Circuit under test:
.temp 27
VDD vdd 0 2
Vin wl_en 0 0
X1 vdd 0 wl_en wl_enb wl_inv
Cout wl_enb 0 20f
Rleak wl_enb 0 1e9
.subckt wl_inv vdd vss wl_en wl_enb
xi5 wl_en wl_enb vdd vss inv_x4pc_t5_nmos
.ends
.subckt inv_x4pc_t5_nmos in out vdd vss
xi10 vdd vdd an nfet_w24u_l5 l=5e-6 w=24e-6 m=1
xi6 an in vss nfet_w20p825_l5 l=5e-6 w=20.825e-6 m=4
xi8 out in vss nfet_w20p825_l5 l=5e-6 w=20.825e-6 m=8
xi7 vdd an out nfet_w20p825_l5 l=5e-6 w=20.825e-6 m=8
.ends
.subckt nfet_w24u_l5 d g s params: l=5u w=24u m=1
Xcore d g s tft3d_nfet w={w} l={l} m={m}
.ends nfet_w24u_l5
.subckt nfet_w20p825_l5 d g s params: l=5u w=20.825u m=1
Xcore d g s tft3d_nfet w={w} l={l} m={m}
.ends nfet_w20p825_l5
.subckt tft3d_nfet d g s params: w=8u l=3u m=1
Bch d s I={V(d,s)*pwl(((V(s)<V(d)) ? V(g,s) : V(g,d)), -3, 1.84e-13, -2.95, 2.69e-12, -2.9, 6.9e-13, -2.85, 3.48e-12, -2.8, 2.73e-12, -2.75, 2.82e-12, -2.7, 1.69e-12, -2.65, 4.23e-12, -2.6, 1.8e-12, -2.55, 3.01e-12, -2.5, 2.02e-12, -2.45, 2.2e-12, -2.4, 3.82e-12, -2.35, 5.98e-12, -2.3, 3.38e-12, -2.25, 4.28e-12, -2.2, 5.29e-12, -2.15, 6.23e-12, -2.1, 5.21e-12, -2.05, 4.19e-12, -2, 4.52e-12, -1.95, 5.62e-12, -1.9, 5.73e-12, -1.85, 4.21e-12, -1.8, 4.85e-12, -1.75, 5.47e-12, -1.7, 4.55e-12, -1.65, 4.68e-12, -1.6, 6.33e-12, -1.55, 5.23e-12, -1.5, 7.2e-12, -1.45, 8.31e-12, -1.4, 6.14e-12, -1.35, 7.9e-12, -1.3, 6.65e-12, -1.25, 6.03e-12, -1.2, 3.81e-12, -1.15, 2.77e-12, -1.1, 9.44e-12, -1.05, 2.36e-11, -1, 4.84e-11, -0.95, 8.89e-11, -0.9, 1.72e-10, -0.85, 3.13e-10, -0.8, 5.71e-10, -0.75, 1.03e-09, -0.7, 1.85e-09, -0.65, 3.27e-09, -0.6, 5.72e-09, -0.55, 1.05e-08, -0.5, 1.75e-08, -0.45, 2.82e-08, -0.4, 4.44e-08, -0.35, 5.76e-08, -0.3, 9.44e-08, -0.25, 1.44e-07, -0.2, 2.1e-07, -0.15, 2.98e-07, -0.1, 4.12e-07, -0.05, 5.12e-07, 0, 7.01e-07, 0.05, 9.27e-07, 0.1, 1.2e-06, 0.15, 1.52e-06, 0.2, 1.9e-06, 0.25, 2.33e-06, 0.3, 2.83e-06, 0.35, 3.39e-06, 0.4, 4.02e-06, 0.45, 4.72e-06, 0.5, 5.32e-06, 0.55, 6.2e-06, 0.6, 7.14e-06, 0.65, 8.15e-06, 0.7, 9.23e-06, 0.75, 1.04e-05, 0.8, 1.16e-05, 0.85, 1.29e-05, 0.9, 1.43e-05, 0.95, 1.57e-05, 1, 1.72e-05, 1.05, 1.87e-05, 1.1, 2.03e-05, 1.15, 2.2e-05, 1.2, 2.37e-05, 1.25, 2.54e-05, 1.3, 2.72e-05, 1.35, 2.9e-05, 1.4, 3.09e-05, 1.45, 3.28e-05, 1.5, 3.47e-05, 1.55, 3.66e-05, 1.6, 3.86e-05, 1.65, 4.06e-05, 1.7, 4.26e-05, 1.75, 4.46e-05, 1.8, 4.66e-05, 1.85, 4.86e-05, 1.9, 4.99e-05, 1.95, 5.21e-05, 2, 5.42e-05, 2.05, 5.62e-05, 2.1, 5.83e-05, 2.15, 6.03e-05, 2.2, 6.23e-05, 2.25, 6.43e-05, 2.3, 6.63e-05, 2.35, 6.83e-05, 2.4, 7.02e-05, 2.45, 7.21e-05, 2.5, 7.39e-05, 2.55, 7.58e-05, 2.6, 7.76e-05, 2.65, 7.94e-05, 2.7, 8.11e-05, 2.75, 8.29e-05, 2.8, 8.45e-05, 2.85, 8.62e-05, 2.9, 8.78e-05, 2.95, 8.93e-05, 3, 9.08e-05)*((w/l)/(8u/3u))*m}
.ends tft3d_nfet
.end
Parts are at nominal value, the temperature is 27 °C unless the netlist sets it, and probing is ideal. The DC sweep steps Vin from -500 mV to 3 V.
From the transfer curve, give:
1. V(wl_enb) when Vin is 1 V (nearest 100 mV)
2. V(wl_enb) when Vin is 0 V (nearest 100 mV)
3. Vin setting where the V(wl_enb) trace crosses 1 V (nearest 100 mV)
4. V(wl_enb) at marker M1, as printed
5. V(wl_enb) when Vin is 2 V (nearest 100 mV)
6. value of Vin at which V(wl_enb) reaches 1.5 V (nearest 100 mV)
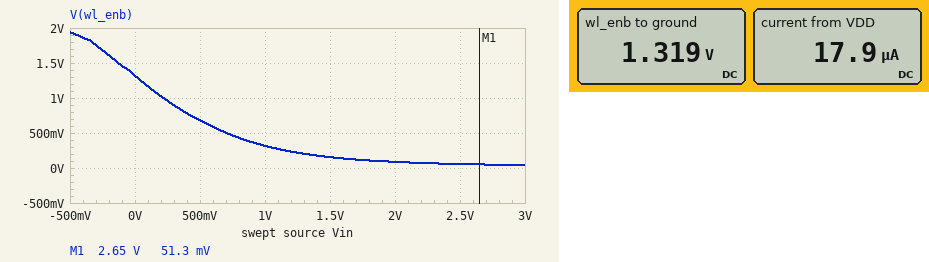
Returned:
300 mV
1.3 V
200 mV
51.3 mV
100 mV
-100 mV
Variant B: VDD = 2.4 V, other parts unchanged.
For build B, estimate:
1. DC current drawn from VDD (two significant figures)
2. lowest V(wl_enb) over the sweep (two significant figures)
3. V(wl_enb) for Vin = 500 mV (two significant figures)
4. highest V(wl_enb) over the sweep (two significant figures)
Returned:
22 µA
70 mV
930 mV
2.3 V
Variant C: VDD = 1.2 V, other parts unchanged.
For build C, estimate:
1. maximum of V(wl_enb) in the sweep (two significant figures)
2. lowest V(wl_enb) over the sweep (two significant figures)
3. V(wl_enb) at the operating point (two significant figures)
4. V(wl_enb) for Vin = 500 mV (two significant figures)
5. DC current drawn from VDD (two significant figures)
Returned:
1.2 V
13 mV
710 mV
280 mV
9.6 µA
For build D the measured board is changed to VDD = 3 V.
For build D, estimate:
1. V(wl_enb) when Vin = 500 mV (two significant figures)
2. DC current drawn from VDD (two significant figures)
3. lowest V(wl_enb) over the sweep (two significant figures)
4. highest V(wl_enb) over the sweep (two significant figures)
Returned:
1.3 V
29 µA
140 mV
2.9 V
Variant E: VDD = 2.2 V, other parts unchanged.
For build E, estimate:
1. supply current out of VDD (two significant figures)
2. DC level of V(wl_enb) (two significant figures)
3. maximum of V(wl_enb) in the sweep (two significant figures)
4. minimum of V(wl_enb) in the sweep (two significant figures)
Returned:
20 µA
1.5 V
2.1 V
54 mV
